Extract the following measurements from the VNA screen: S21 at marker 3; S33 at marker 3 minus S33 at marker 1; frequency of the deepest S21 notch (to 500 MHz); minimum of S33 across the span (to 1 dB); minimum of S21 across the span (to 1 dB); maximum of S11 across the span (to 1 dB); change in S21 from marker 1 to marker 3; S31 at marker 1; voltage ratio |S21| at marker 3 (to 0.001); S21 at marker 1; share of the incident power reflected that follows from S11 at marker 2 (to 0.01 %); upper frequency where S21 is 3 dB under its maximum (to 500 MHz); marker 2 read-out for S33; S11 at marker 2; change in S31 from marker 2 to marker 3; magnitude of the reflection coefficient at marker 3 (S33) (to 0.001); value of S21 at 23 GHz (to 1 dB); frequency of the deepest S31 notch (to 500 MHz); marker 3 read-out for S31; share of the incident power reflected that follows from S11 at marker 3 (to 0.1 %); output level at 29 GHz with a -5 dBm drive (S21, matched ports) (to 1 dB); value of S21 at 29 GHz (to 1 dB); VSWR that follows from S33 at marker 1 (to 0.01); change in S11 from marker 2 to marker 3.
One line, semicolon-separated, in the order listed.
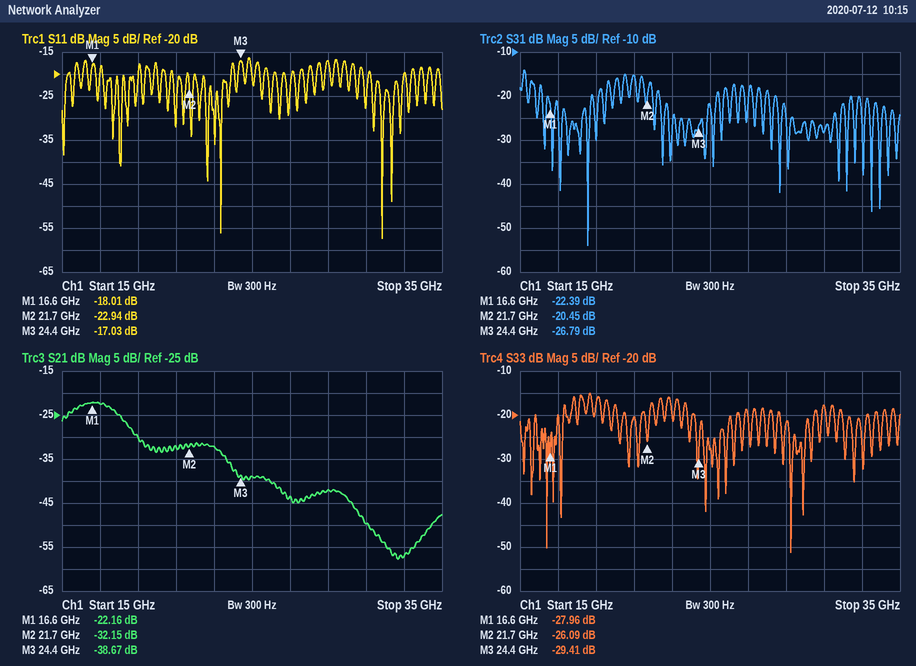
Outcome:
-38.67 dB; -1.45 dB; 32.5 GHz; -51 dB; -58 dB; -16 dB; -16.51 dB; -22.39 dB; 0.012; -22.16 dB; 0.51 %; 18.0 GHz; -26.09 dB; -22.94 dB; -6.34 dB; 0.034; -32 dB; 18.5 GHz; -26.79 dB; 2.0 %; -47 dBm; -42 dB; 1.08; 5.91 dB
